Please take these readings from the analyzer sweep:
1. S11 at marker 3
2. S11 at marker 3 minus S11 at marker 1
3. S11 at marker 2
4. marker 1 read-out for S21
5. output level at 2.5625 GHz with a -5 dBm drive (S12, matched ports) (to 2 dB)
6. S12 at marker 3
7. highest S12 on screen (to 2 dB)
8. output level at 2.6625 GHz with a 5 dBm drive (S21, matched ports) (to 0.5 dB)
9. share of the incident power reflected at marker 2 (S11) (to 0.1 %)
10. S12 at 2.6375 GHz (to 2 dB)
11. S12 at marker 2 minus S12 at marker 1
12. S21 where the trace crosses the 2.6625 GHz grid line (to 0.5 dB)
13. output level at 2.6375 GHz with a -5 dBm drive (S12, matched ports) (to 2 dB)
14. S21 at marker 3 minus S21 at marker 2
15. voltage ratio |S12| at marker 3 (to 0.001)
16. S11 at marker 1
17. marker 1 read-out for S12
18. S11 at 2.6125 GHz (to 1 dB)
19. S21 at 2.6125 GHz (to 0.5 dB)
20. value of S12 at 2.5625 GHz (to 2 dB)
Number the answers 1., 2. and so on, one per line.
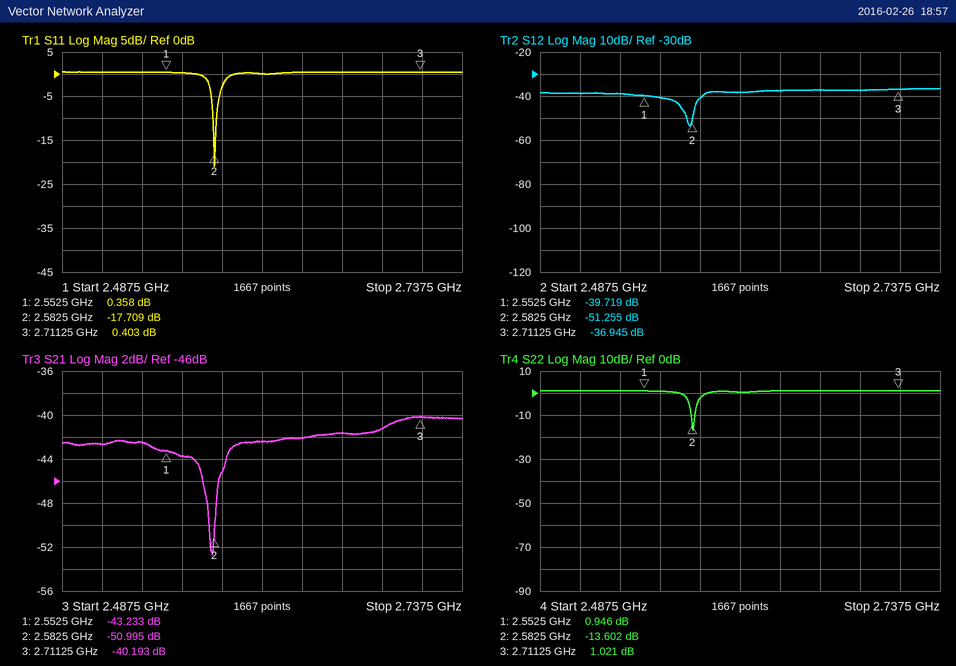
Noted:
1. 0.403 dB
2. 0.045 dB
3. -17.709 dB
4. -43.233 dB
5. -46 dBm
6. -36.945 dB
7. -36 dB
8. -36.5 dBm
9. 1.7 %
10. -38 dB
11. -11.536 dB
12. -41.5 dB
13. -42 dBm
14. 10.802 dB
15. 0.014
16. 0.358 dB
17. -39.719 dB
18. 0 dB
19. -42.5 dB
20. -40 dB
